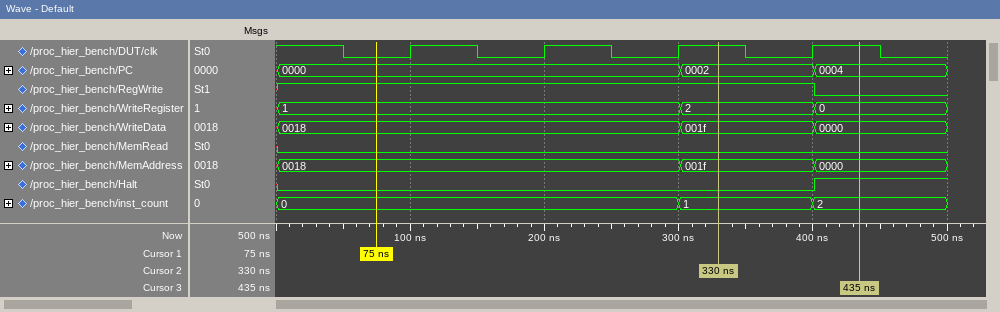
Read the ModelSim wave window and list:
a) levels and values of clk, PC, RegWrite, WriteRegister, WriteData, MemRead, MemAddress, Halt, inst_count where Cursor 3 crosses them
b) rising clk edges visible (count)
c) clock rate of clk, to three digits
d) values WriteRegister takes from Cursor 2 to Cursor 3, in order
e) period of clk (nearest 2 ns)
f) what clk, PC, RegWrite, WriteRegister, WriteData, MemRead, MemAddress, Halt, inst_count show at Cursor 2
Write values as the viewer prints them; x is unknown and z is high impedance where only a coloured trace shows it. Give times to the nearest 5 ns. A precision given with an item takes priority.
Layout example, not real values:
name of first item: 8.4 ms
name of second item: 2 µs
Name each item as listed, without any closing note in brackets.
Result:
levels and values of clk, PC, RegWrite, WriteRegister, WriteData, MemRead, MemAddress, Halt, inst_count where Cursor 3 crosses them: clk=1, PC=0004, RegWrite=0, WriteRegister=0, WriteData=0000, MemRead=0, MemAddress=0000, Halt=1, inst_count=2
rising clk edges visible: 4
clock rate of clk, to three digits: 10.0 MHz
values WriteRegister takes from Cursor 2 to Cursor 3, in order: 2, 0
period of clk: 100 ns
what clk, PC, RegWrite, WriteRegister, WriteData, MemRead, MemAddress, Halt, inst_count show at Cursor 2: clk=1, PC=0002, RegWrite=1, WriteRegister=2, WriteData=001f, MemRead=0, MemAddress=001f, Halt=0, inst_count=1
